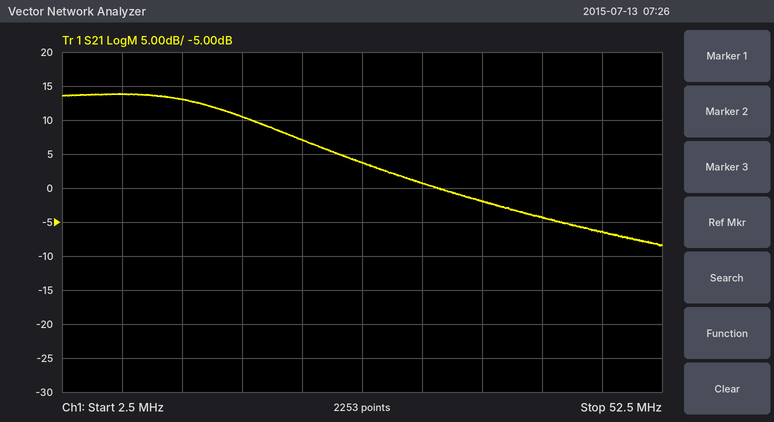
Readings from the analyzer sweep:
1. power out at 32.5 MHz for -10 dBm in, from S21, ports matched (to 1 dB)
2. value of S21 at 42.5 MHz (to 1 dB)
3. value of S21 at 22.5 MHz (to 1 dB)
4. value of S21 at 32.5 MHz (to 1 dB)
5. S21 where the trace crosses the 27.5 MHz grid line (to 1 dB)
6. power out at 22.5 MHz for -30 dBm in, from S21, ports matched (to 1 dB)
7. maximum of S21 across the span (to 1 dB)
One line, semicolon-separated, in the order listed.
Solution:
-9 dBm; -4 dB; 7 dB; 1 dB; 4 dB; -23 dBm; 14 dB
